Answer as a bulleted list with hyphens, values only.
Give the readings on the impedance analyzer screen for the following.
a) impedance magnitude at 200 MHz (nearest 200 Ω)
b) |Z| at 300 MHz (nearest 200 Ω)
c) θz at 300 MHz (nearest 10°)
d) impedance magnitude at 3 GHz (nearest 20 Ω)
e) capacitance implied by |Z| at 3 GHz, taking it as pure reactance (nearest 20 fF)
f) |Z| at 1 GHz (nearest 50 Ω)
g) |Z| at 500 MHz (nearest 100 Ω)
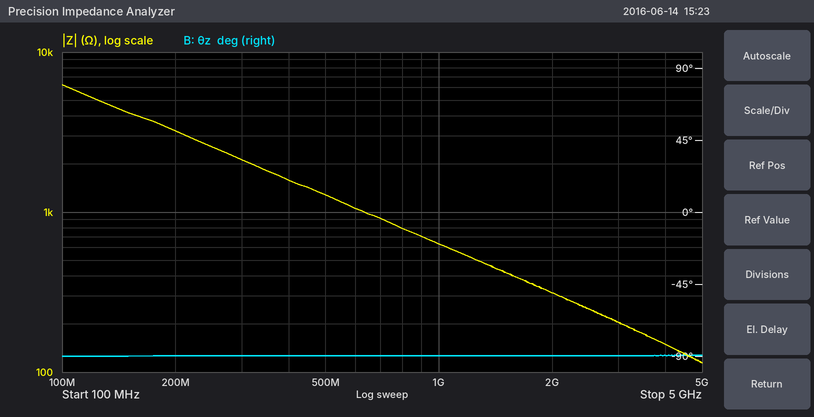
- 3.2 kΩ
- 2.2 kΩ
- -90°
- 200 Ω
- 260 fF
- 650 Ω
- 1.3 kΩ
